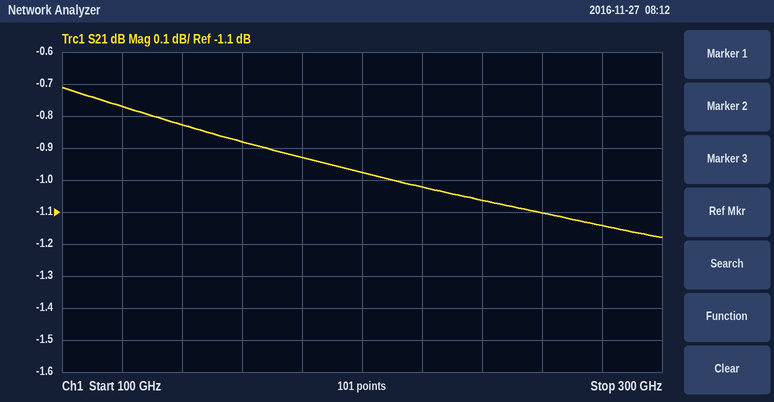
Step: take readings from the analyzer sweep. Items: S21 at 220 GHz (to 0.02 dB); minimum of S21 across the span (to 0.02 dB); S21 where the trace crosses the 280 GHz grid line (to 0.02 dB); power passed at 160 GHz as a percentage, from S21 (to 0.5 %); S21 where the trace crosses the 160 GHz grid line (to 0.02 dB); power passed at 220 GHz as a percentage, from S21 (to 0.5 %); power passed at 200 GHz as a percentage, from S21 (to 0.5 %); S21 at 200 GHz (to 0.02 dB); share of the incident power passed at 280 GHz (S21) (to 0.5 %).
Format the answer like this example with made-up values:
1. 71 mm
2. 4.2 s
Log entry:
1. -1.02 dB
2. -1.18 dB
3. -1.14 dB
4. 81.5 %
5. -0.88 dB
6. 79.0 %
7. 80.0 %
8. -0.98 dB
9. 77.0 %
